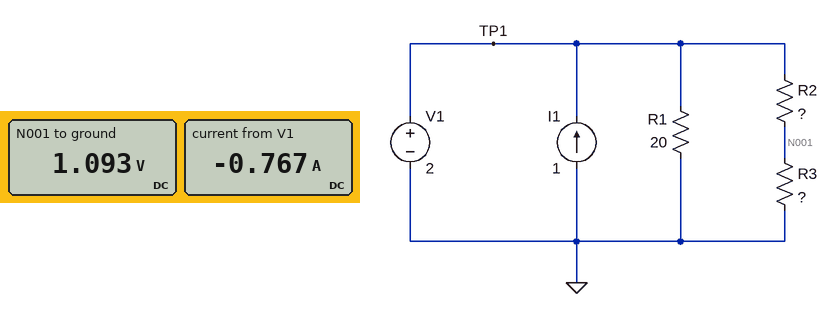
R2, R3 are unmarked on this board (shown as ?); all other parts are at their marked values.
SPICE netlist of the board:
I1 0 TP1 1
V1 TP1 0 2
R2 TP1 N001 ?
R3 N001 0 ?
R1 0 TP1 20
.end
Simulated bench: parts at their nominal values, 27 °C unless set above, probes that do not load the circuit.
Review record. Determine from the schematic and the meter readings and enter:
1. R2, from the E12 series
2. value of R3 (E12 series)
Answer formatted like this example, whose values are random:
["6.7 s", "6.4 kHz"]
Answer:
["6.8 Ω", "8.2 Ω"]
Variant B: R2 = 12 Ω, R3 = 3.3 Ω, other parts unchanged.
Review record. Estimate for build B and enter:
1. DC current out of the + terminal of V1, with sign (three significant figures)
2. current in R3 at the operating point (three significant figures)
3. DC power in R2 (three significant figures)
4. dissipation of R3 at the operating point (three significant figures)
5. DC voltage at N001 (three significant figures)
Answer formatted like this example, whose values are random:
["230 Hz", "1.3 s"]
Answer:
["-769 mA", "131 mA", "205 mW", "56.4 mW", "431 mV"]
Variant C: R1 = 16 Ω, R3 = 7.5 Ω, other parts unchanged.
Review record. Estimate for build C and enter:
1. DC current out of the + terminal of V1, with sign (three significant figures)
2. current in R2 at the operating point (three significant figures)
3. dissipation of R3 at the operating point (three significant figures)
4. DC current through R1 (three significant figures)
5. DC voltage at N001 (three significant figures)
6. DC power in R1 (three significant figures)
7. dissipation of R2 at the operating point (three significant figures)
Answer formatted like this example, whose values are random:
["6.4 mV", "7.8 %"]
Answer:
["-735 mA", "140 mA", "147 mW", "125 mA", "1.05 V", "250 mW", "133 mW"]
